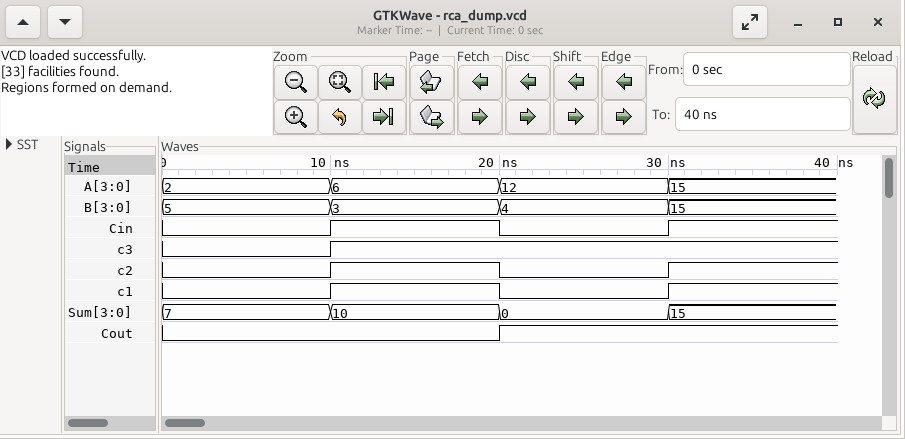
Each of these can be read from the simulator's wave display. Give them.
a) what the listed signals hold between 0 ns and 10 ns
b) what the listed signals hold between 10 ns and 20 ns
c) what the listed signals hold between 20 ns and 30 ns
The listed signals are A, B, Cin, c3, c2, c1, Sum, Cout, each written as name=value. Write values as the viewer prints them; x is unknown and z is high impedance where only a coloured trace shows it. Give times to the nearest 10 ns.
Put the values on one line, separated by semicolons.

A=2, B=5, Cin=0, c3=0, c2=0, c1=0, Sum=7, Cout=0; A=6, B=3, Cin=1, c3=1, c2=1, c1=1, Sum=10, Cout=0; A=12, B=4, Cin=0, c3=1, c2=0, c1=0, Sum=0, Cout=1
